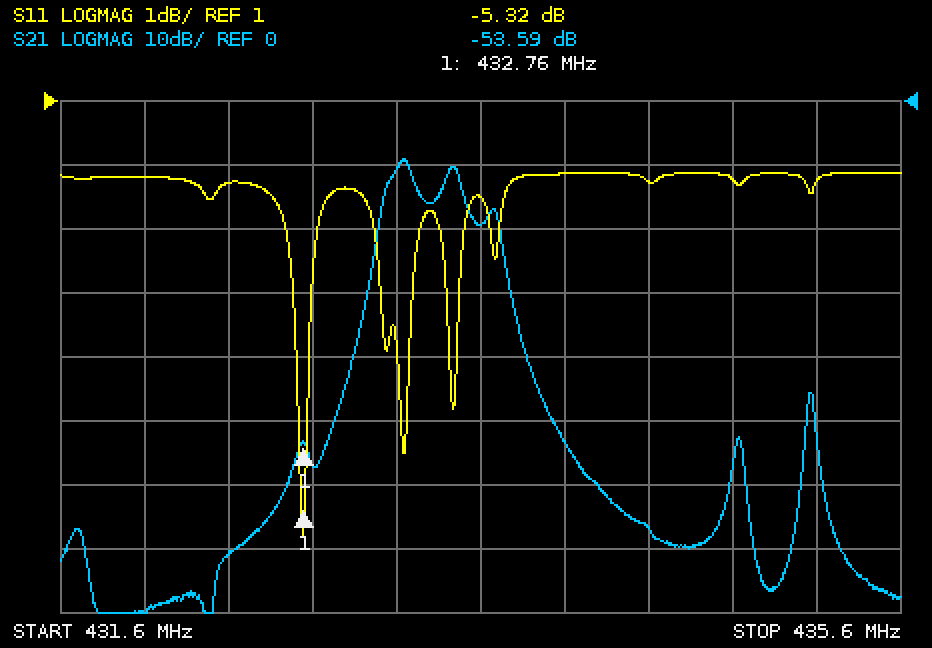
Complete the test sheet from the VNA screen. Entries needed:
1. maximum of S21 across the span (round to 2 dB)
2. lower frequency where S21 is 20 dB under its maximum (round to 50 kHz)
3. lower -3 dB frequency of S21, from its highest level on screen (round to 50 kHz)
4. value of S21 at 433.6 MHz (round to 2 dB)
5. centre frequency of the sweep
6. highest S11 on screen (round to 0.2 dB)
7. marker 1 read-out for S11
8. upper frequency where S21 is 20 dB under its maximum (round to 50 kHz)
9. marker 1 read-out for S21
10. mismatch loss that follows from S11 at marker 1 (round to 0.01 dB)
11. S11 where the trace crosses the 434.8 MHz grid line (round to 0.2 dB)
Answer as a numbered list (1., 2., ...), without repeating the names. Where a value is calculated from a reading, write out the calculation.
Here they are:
1. -10 dB
2. 433.05 MHz
3. 433.15 MHz
4. -20 dB
5. 433.6 MHz
6. -0.2 dB
7. -5.32 dB
8. 433.75 MHz
9. -53.59 dB
10. −10 log10(1 − 10^(-5.32/10)) ≈ 1.51 dB
11. -0.2 dB
